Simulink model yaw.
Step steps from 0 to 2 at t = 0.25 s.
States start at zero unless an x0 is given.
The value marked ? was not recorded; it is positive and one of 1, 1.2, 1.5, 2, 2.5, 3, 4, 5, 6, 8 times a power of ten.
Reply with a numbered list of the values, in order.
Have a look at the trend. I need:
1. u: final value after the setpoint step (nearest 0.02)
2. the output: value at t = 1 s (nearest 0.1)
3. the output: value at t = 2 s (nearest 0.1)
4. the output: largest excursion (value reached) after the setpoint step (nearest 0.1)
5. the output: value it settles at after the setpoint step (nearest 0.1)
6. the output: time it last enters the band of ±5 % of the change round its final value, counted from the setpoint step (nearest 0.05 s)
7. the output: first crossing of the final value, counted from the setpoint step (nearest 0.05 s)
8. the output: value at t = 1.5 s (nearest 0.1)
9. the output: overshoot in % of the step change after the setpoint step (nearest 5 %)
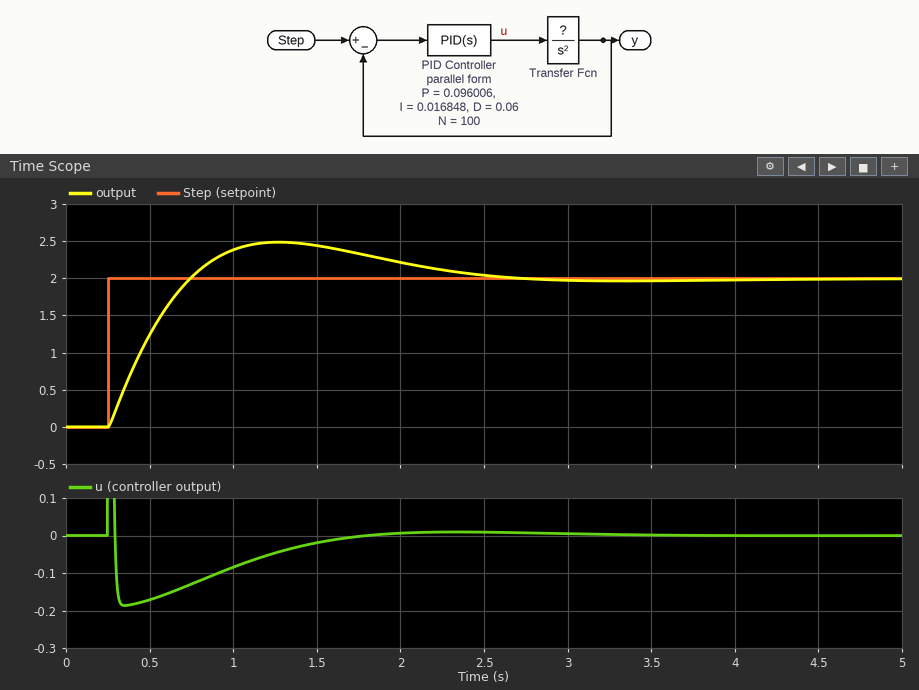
1. 0.00
2. 2.4
3. 2.2
4. 2.5
5. 2.0
6. 2.05 s
7. 0.50 s
8. 2.4
9. 25 %
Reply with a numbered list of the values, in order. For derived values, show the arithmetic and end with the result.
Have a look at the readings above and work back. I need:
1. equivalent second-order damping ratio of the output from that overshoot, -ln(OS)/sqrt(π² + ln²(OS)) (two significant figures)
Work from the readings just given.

1. ln(0.25) = -1.386; 1.386 / sqrt(9.870 + 1.922) = 0.40
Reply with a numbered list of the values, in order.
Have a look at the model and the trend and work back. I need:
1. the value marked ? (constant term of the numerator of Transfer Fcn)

1. 50
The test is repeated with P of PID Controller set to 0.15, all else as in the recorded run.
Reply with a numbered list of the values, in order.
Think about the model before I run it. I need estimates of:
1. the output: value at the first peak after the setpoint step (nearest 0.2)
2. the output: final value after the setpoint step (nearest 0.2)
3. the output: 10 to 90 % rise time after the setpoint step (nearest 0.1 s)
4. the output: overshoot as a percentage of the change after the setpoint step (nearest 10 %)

1. 2.6
2. 2.0
3. 0.3 s
4. 30 %
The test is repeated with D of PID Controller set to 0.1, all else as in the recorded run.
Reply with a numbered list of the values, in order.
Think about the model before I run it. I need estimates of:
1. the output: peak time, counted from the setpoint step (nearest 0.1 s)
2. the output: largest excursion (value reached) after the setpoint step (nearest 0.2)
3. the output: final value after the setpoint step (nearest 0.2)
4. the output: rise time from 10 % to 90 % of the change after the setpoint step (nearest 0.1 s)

1. 0.9 s
2. 2.2
3. 2.0
4. 0.3 s
